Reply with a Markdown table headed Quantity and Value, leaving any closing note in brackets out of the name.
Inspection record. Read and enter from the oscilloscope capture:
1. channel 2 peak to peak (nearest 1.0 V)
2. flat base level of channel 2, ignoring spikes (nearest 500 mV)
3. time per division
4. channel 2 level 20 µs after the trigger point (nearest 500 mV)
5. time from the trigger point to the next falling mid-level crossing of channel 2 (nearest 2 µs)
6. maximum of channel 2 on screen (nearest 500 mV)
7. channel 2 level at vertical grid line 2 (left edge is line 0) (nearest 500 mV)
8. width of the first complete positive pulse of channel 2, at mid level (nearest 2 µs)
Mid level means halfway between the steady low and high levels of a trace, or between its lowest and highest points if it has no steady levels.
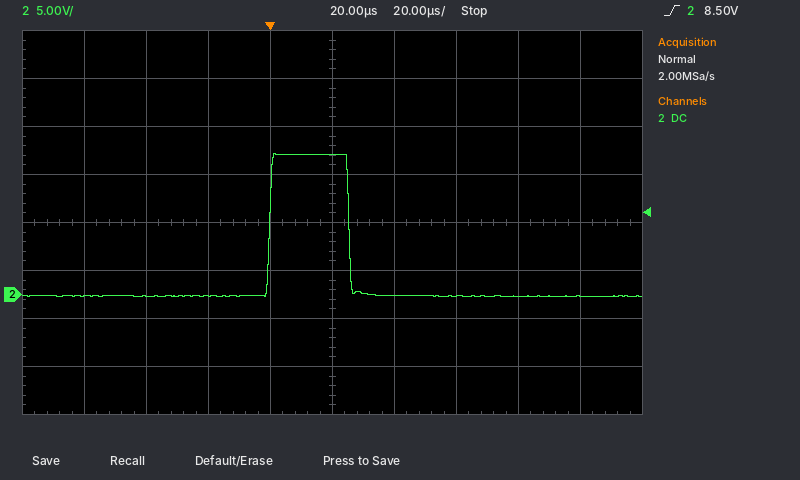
| Quantity | Value |
|---|---|
| channel 2 peak to peak | 15.0 V |
| flat base level of channel 2, ignoring spikes | 0.0 V |
| time per division | 20 µs |
| channel 2 level 20 µs after the trigger point | 14.5 V |
| time from the trigger point to the next falling mid-level crossing of channel 2 | 26 µs |
| maximum of channel 2 on screen | 14.5 V |
| channel 2 level at vertical grid line 2 (left edge is line 0) | 0.0 V |
| width of the first complete positive pulse of channel 2, at mid level | 26 µs |
